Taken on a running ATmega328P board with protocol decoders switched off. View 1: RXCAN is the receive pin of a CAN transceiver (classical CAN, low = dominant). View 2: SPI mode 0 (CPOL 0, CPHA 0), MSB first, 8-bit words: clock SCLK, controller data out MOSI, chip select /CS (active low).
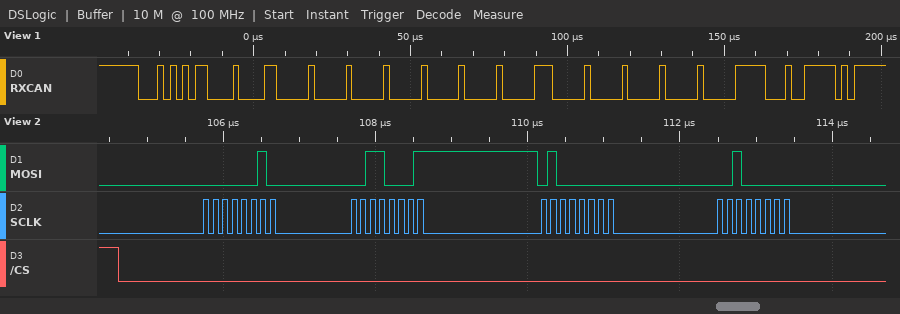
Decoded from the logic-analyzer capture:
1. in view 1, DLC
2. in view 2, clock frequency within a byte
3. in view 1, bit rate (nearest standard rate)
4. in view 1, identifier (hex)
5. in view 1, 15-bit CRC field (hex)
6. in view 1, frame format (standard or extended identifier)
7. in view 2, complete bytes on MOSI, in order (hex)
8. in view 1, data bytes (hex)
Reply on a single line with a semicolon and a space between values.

8; 8 MHz; 500 kbit/s; 0x156; 0x3C9F; standard; 02 31 40 20; 60 00 00 00 03 00 00 00
